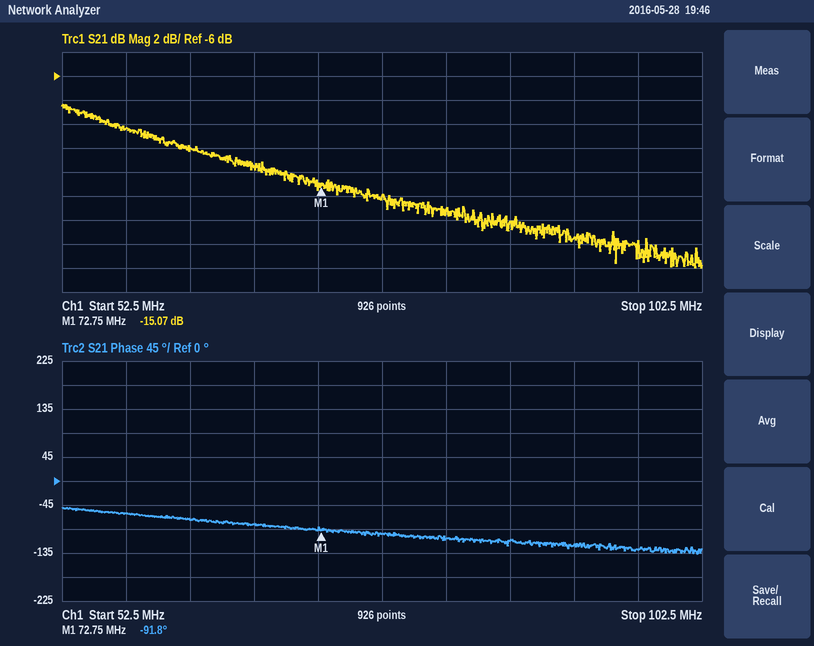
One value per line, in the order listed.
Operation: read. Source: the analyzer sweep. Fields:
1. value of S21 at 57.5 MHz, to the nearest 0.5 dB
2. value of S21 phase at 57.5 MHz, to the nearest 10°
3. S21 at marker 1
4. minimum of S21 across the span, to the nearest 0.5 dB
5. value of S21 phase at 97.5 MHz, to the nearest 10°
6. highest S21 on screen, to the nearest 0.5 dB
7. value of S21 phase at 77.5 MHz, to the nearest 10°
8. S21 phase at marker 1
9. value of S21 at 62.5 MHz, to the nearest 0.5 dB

-10.5 dB
-60°
-15.07 dB
-22.0 dB
-130°
-8.5 dB
-100°
-91.8°
-12.0 dB
